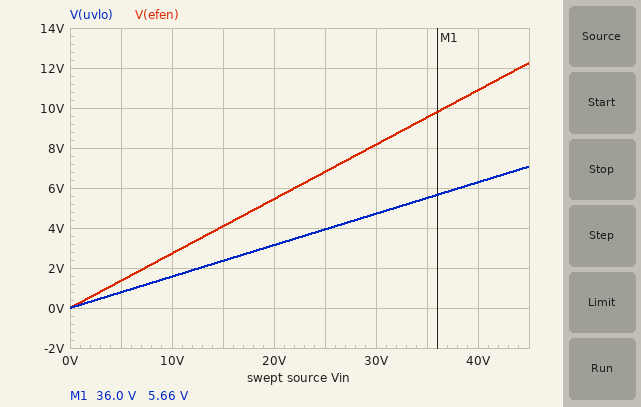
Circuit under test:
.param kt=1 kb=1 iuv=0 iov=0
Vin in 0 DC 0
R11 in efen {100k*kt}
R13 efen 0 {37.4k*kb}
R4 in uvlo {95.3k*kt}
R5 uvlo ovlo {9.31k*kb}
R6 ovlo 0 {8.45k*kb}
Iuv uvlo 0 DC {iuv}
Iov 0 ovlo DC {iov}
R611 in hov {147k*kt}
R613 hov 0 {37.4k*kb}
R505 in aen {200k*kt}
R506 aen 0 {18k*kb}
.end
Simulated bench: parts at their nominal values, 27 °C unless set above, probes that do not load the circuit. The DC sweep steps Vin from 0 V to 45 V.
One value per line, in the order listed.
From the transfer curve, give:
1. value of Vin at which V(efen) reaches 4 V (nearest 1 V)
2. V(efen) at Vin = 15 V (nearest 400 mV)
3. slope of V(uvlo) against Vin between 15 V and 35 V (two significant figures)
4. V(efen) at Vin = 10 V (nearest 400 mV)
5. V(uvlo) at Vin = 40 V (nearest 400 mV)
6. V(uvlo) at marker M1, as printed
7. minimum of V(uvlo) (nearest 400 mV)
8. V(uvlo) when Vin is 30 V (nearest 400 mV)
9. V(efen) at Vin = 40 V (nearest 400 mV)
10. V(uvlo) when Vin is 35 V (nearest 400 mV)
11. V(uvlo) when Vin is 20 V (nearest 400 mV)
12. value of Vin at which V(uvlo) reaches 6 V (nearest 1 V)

15 V
4.0 V
0.16 V/V
2.8 V
6.4 V
5.66 V
0 V
4.8 V
10.8 V
5.6 V
3.2 V
38 V
